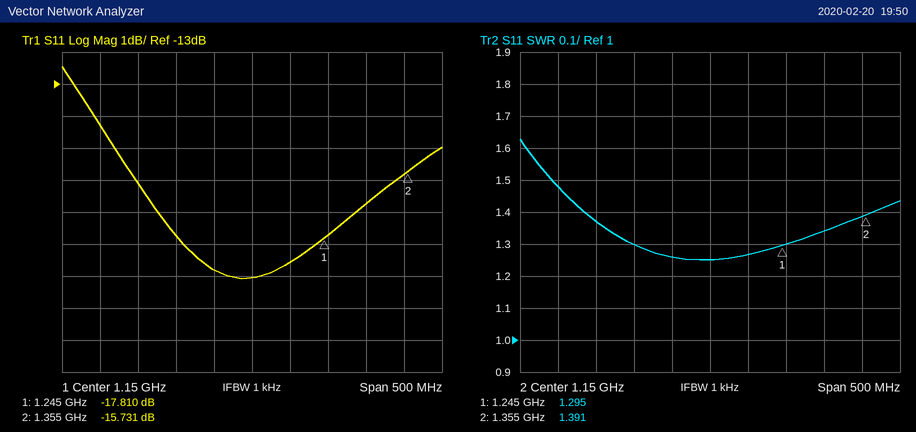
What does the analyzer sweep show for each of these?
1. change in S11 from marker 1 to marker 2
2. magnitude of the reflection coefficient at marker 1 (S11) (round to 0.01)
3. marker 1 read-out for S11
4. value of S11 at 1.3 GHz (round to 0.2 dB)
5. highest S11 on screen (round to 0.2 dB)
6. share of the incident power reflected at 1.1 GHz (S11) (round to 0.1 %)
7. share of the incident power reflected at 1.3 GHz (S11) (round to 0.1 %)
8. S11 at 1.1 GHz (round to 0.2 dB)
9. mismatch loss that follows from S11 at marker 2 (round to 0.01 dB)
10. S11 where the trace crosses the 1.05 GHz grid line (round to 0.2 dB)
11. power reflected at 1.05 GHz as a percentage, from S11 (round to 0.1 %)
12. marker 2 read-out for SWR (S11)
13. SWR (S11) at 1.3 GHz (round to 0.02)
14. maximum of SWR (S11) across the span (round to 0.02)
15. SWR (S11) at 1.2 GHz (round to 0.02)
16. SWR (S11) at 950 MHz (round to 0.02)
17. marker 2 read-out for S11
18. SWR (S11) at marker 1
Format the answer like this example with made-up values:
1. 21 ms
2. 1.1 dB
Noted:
1. 2.079 dB
2. 0.13
3. -17.810 dB
4. -16.8 dB
5. -12.4 dB
6. 1.3 %
7. 2.1 %
8. -18.8 dB
9. 0.12 dB
10. -17.8 dB
11. 1.7 %
12. 1.391
13. 1.34
14. 1.62
15. 1.26
16. 1.48
17. -15.731 dB
18. 1.295
